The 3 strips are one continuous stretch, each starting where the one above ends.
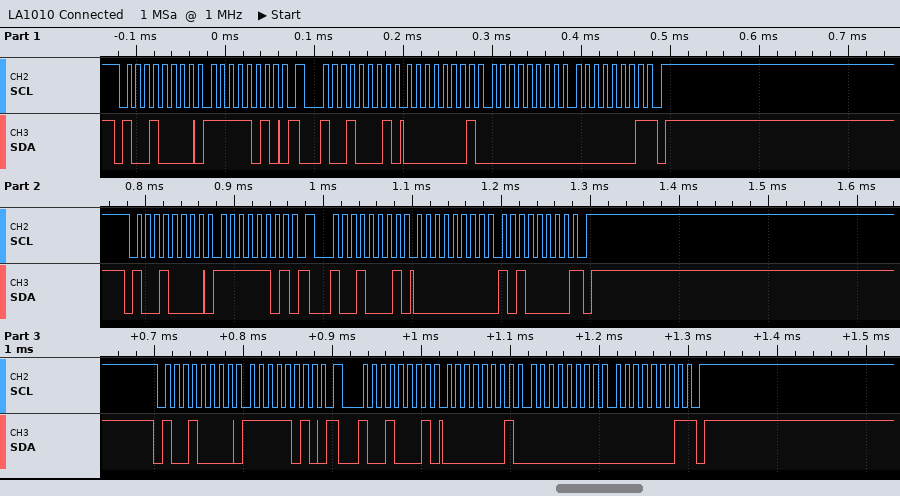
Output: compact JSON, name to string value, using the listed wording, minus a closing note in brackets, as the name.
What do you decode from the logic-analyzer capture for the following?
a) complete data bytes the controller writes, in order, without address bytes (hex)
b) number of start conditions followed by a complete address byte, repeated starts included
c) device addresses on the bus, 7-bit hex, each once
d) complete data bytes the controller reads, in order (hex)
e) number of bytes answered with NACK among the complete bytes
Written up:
{"complete data bytes the controller writes, in order, without address bytes": "FA FD FA", "number of start conditions followed by a complete address byte, repeated starts included": "6", "device addresses on the bus, 7-bit hex, each once": "0x48", "complete data bytes the controller reads, in order": "01 00 01 00 A0 01 00 01", "number of bytes answered with NACK among the complete bytes": "3"}
